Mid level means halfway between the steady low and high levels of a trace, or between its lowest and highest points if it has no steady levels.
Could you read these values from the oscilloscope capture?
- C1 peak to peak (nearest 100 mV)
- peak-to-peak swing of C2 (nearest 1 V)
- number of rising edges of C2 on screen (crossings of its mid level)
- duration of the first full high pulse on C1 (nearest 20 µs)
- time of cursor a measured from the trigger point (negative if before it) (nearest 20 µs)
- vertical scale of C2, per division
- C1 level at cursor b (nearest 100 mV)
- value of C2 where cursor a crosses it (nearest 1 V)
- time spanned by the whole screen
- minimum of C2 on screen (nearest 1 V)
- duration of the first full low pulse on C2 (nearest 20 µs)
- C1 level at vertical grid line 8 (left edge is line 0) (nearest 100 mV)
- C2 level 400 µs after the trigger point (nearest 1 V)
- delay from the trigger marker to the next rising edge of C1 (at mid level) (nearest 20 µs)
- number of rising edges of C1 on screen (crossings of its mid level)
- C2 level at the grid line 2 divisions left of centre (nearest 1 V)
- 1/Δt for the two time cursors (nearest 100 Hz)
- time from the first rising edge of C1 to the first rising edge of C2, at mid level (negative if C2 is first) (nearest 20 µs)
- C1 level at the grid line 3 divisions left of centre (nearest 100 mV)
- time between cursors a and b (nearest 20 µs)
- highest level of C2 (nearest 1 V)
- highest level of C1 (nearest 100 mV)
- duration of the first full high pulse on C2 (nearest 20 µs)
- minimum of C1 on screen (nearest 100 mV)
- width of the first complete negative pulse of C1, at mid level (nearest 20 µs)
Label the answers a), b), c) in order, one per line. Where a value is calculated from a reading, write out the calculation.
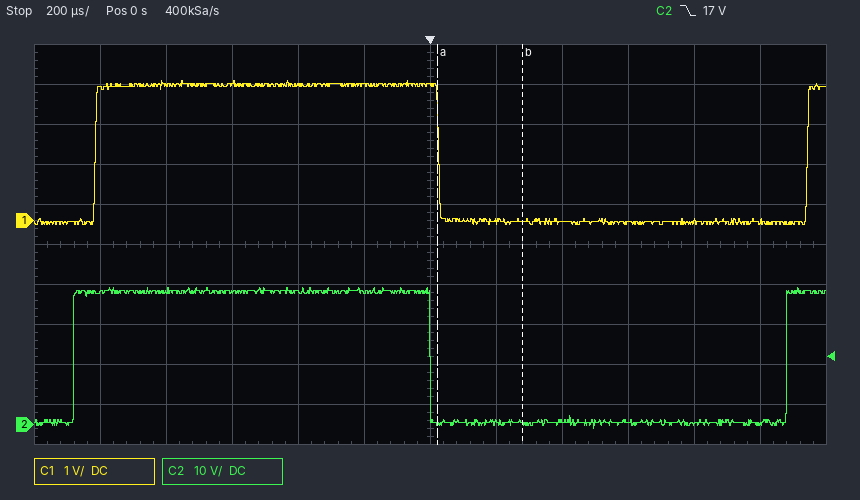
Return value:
a) 3.5 V − (-100 mV) = 3.6 V
b) 34 V − (-1 V) = 35 V
c) 2
d) 1.04 ms
e) +20 µs
f) 10 V
g) 0.0 V
h) 0 V
i) 2.4 ms
j) -1 V
k) 1.08 ms
l) 0.0 V
m) 1 V
n) 1.14 ms
o) 2
p) 33 V
q) 1 / 260 µs ≈ 3.8 kHz
r) -60 µs
s) 3.4 V
t) 260 µs
u) 34 V
v) 3.5 V
w) 1.08 ms
x) -100 mV
y) 1.12 ms
